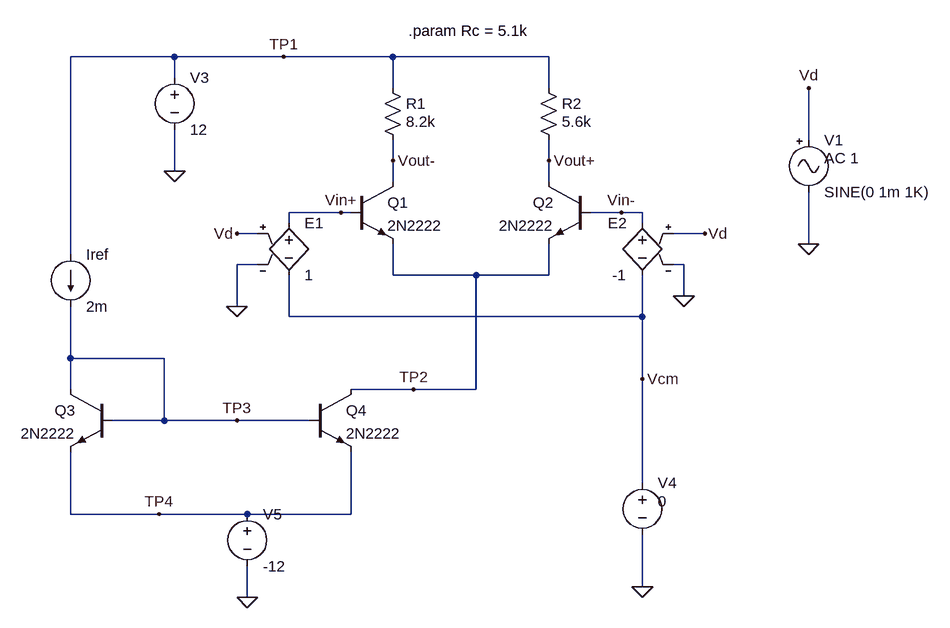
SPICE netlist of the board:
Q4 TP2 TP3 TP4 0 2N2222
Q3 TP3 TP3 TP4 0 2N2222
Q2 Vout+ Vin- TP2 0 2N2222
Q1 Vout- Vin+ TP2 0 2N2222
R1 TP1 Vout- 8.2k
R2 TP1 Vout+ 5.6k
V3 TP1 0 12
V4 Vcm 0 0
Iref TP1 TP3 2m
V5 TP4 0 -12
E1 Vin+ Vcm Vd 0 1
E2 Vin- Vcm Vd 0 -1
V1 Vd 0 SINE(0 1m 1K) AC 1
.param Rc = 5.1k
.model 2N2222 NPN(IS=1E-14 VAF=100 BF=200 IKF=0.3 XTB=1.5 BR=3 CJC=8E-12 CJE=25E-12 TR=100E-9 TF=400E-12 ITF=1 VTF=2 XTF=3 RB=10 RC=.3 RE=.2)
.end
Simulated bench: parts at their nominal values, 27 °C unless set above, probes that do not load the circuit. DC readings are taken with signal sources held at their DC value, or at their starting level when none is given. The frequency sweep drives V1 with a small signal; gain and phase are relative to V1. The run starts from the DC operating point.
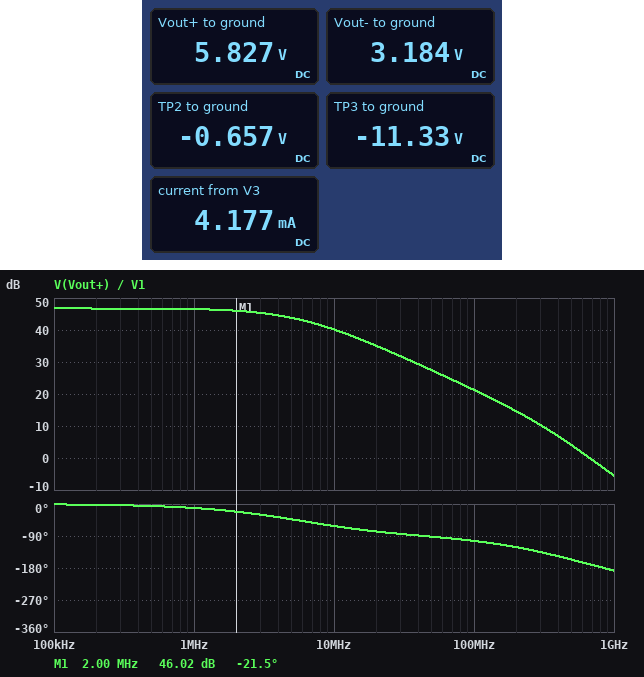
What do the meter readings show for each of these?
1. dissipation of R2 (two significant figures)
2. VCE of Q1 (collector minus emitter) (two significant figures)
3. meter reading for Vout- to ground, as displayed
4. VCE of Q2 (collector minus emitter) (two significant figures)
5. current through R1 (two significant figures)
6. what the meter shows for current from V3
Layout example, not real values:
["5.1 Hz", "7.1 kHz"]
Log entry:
["6.8 mW", "3.8 V", "3.184 V", "6.5 V", "1.1 mA", "4.177 mA"]
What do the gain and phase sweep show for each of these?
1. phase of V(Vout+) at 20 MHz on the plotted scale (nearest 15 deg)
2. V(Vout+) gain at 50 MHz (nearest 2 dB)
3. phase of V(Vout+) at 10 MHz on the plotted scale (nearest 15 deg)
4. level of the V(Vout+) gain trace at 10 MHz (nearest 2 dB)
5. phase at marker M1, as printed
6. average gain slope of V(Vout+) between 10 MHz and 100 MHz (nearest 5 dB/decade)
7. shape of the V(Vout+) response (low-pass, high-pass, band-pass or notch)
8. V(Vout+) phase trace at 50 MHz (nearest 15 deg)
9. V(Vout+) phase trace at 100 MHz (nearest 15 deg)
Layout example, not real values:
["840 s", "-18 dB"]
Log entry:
["-75 deg", "28 dB", "-60 deg", "40 dB", "-21.5 deg", "-20 dB/decade", "low-pass", "-90 deg", "-105 deg"]
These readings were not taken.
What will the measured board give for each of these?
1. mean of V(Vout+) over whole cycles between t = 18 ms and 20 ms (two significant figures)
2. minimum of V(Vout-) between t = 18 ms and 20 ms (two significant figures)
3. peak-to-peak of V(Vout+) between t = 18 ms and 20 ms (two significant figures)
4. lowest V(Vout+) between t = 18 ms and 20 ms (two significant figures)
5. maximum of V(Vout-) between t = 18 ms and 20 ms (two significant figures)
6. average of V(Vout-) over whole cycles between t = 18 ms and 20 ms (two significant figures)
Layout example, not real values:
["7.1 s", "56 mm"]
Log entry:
["5.8 V", "2.9 V", "430 mV", "5.6 V", "3.5 V", "3.2 V"]
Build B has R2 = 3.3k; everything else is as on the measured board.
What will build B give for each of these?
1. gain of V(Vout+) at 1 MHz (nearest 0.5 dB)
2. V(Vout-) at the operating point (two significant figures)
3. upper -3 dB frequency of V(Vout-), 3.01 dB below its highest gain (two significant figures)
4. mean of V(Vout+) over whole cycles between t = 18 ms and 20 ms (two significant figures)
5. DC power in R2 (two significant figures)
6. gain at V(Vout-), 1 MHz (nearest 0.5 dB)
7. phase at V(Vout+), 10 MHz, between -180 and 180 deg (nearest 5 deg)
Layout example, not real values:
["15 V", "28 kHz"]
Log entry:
["42.0 dB", "3.3 V", "3.5 MHz", "8.3 V", "4.1 mW", "50.0 dB", "-45 deg"]
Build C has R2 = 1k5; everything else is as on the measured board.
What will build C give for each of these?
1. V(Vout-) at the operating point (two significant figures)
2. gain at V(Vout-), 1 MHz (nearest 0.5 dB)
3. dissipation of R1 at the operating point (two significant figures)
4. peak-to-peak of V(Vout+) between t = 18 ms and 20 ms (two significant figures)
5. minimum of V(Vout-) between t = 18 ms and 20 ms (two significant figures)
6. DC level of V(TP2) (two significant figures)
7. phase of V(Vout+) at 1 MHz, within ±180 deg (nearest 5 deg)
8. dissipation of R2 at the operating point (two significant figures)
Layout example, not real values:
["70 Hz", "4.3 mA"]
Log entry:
["3.4 V", "50.0 dB", "9.1 mW", "120 mV", "3.0 V", "-660 mV", "-5 deg", "1.9 mW"]
